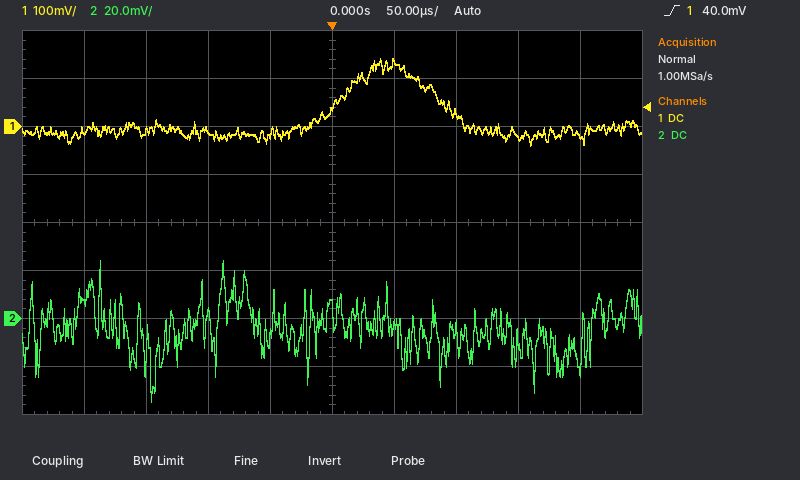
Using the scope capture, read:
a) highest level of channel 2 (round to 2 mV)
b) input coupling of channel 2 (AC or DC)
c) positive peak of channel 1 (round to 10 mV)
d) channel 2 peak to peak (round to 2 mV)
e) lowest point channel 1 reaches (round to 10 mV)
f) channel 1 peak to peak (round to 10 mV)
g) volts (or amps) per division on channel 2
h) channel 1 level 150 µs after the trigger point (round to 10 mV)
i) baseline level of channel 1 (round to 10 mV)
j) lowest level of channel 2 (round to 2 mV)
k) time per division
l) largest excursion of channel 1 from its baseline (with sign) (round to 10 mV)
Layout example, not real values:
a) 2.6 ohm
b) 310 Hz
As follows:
a) 24 mV
b) DC
c) 140 mV
d) 58 mV
e) -40 mV
f) 180 mV
g) 20 mV
h) -20 mV
i) -10 mV
j) -34 mV
k) 50 µs
l) +150 mV
